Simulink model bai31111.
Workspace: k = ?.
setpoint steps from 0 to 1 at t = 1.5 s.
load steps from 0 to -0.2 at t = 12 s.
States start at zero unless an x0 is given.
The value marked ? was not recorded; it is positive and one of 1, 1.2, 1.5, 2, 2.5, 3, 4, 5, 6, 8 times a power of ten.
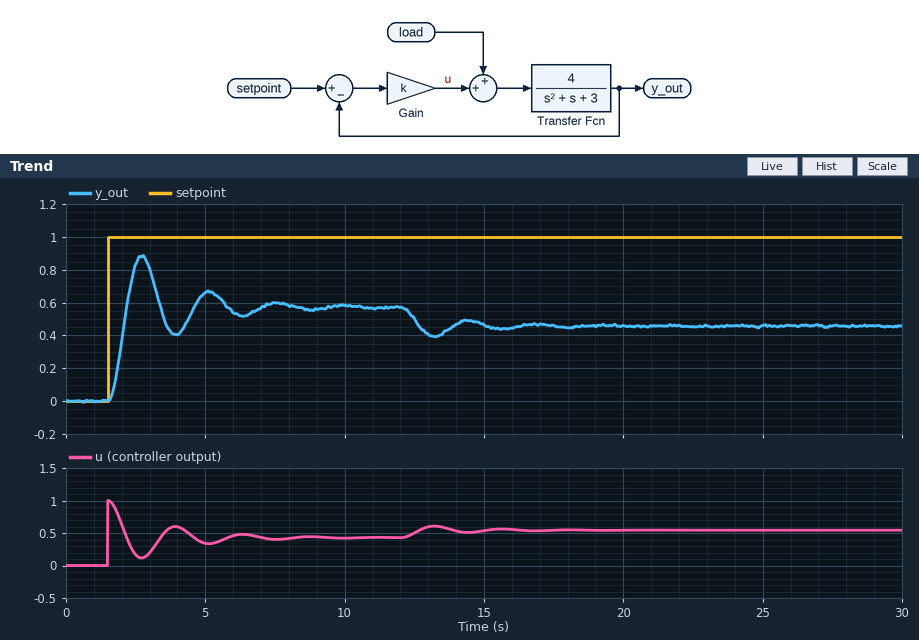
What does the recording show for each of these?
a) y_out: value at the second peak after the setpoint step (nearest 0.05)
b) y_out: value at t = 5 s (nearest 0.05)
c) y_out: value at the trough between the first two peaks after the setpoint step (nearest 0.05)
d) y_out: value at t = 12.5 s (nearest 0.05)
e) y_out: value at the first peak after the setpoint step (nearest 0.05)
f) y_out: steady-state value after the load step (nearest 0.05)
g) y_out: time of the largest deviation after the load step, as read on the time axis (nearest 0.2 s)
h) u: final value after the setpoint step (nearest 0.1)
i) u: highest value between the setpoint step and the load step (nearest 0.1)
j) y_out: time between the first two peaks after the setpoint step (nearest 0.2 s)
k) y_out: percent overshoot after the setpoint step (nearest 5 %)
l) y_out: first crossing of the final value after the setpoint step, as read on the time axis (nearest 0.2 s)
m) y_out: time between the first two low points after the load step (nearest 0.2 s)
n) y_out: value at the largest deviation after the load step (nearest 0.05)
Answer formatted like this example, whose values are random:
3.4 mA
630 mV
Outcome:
0.65
0.65
0.40
0.50
0.90
0.45
13.2 s
0.4
1.0
2.4 s
55 %
2.2 s
2.4 s
0.40
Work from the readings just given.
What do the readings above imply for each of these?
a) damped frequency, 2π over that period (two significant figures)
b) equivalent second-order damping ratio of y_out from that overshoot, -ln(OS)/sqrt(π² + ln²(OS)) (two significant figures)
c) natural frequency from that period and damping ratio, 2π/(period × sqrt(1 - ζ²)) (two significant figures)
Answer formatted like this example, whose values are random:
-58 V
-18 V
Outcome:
2.6 rad/s
0.19
2.7 rad/s
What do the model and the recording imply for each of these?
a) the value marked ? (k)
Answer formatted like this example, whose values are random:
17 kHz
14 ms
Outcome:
1
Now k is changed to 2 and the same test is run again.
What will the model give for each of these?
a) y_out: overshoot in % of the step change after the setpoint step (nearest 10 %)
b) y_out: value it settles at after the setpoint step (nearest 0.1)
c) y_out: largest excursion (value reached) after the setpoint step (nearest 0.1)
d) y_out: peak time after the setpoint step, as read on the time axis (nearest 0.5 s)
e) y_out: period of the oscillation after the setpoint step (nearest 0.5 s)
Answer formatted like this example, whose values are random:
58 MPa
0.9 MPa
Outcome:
60 %
0.7
1.2
2.5 s
2.0 s
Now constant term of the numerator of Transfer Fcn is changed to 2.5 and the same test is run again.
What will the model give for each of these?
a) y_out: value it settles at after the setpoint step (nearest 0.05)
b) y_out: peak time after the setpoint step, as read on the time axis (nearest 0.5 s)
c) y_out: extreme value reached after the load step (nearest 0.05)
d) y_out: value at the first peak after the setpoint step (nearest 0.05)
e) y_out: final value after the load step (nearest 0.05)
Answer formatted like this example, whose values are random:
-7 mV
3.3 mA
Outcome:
0.45
3.0 s
0.30
0.70
0.35
